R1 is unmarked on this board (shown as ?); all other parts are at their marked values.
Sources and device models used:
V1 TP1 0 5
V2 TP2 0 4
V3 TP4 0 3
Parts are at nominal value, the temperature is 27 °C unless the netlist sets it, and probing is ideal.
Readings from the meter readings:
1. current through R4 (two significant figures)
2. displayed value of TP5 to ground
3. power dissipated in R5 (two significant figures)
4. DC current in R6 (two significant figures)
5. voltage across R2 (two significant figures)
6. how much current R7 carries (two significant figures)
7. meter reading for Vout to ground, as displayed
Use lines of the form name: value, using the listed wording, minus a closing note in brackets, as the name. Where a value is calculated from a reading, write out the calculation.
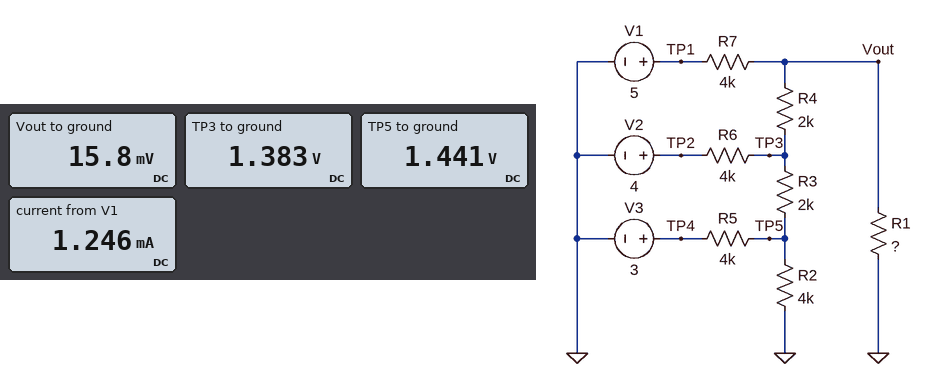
current through R4: (1.383 V - 15.8 mV) / 2 kΩ = 680 µA
displayed value of TP5 to ground: 1.441 V
power dissipated in R5: (3 V - 1.441 V)^2 / 4 kΩ = 610 µW
DC current in R6: (4 V - 1.383 V) / 4 kΩ = 650 µA
voltage across R2: 1.441 V = 1.4 V
how much current R7 carries: (5 V - 15.8 mV) / 4 kΩ = 1.2 mA
meter reading for Vout to ground, as displayed: 15.8 mV
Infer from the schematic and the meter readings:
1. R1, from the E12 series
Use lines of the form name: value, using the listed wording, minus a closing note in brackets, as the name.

R1, from the E12 series: 8.2 Ω
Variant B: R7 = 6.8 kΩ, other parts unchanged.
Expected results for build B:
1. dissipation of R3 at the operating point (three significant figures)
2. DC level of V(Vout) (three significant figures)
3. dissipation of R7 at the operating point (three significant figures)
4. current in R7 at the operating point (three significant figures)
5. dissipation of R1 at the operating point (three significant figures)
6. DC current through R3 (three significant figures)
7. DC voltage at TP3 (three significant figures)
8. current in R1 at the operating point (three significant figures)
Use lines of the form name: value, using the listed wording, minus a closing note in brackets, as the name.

dissipation of R3 at the operating point: 1.78 µW
DC level of V(Vout): 11.6 mV
dissipation of R7 at the operating point: 3.66 mW
current in R7 at the operating point: 734 µA
dissipation of R1 at the operating point: 16.5 µW
DC current through R3: 29.8 µA
DC voltage at TP3: 1.38 V
current in R1 at the operating point: 1.42 mA
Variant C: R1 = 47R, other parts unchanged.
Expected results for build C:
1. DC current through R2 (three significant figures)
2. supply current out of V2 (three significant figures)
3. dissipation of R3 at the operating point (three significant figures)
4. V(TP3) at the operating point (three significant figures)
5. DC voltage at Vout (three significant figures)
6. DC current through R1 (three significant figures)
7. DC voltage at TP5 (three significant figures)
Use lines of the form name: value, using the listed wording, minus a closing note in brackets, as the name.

DC current through R2: 365 µA
supply current out of V2: 645 µA
dissipation of R3 at the operating point: 810 nW
V(TP3) at the operating point: 1.42 V
DC voltage at Vout: 89.0 mV
DC current through R1: 1.89 mA
DC voltage at TP5: 1.46 V
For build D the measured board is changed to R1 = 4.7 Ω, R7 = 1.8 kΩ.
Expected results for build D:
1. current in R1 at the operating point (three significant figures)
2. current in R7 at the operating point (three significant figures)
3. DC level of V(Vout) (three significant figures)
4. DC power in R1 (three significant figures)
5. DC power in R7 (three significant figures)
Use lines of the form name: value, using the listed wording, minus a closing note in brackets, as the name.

current in R1 at the operating point: 3.45 mA
current in R7 at the operating point: 2.77 mA
DC level of V(Vout): 16.2 mV
DC power in R1: 56.0 µW
DC power in R7: 13.8 mW
